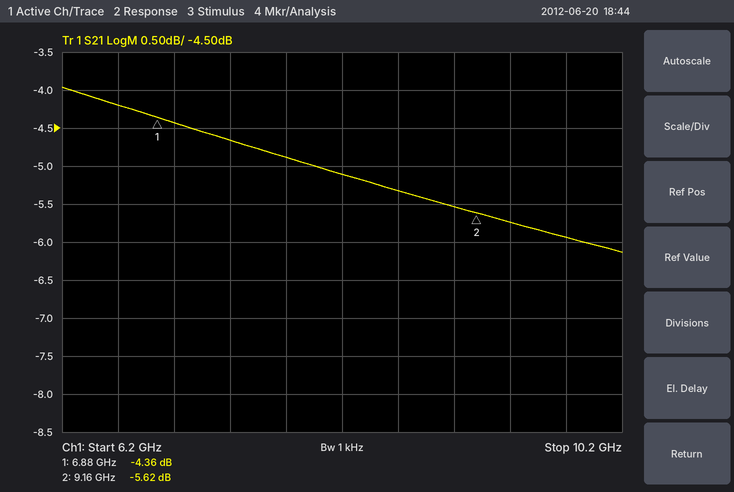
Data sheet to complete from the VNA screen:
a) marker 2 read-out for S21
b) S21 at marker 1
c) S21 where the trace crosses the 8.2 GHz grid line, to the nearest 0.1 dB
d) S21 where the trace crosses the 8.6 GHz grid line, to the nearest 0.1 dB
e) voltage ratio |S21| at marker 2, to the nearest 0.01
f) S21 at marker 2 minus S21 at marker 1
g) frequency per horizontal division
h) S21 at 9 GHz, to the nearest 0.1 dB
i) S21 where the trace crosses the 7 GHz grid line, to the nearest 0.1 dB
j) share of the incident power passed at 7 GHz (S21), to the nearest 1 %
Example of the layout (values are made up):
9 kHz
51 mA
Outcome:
-5.62 dB
-4.36 dB
-5.1 dB
-5.3 dB
0.52
-1.26 dB
400 MHz
-5.5 dB
-4.4 dB
36 %
